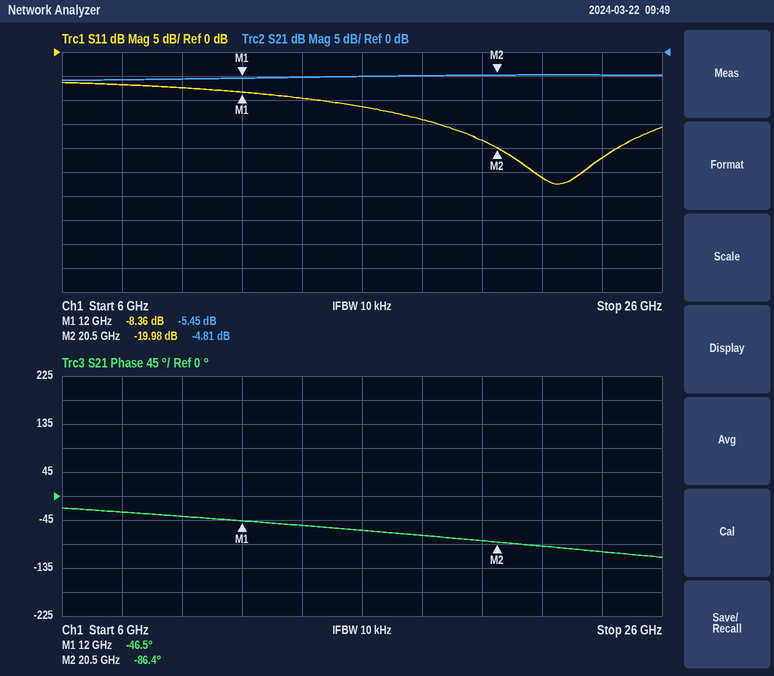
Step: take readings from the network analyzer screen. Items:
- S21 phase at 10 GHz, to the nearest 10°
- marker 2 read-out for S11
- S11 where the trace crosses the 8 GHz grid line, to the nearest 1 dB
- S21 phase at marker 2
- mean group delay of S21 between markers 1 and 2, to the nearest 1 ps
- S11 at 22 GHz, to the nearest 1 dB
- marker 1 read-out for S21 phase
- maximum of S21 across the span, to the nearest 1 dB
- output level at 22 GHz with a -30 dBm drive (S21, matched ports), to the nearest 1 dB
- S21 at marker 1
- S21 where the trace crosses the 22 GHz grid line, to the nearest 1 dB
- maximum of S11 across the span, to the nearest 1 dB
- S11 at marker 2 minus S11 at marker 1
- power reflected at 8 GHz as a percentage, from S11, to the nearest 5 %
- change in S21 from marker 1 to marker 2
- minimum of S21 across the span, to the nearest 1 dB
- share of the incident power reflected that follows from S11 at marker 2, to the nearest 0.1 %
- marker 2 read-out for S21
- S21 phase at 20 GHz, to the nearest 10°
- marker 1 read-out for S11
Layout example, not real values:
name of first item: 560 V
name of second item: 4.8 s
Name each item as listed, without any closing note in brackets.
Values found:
S21 phase at 10 GHz, to the nearest 10°: -40°
marker 2 read-out for S11: -19.98 dB
S11 where the trace crosses the 8 GHz grid line, to the nearest 1 dB: -7 dB
S21 phase at marker 2: -86.4°
mean group delay of S21 between markers 1 and 2, to the nearest 1 ps: 13 ps
S11 at 22 GHz, to the nearest 1 dB: -26 dB
marker 1 read-out for S21 phase: -46.5°
maximum of S21 across the span, to the nearest 1 dB: -5 dB
output level at 22 GHz with a -30 dBm drive (S21, matched ports), to the nearest 1 dB: -35 dBm
S21 at marker 1: -5.45 dB
S21 where the trace crosses the 22 GHz grid line, to the nearest 1 dB: -5 dB
maximum of S11 across the span, to the nearest 1 dB: -6 dB
S11 at marker 2 minus S11 at marker 1: -11.62 dB
power reflected at 8 GHz as a percentage, from S11, to the nearest 5 %: 20 %
change in S21 from marker 1 to marker 2: 0.64 dB
minimum of S21 across the span, to the nearest 1 dB: -6 dB
share of the incident power reflected that follows from S11 at marker 2, to the nearest 0.1 %: 1.0 %
marker 2 read-out for S21: -4.81 dB
S21 phase at 20 GHz, to the nearest 10°: -80°
marker 1 read-out for S11: -8.36 dB
